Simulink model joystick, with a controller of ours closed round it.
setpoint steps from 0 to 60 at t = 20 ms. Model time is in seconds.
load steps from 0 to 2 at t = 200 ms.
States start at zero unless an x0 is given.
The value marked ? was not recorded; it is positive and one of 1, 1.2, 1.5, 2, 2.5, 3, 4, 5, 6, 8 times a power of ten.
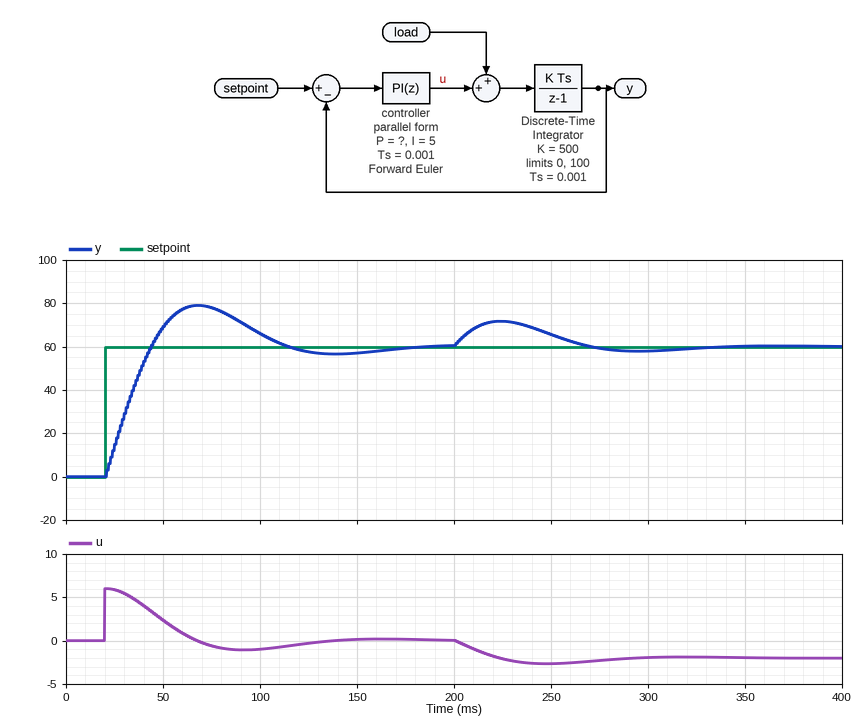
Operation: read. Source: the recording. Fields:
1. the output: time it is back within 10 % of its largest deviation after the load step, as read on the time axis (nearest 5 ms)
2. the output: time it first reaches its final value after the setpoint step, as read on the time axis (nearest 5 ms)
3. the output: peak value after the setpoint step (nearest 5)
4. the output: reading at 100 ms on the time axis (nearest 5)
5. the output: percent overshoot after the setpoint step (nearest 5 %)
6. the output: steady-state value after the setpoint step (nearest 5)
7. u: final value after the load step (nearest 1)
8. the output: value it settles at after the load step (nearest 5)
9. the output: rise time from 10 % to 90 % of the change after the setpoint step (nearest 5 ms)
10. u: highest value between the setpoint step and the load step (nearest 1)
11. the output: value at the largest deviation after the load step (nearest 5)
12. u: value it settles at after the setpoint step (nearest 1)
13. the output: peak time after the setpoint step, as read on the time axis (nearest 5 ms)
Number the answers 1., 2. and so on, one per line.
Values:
1. 320 ms
2. 45 ms
3. 80
4. 65
5. 30 %
6. 60
7. -2
8. 60
9. 20 ms
10. 6
11. 70
12. 0
13. 70 ms
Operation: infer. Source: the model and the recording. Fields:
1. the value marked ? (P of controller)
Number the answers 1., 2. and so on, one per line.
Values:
1. 0.1
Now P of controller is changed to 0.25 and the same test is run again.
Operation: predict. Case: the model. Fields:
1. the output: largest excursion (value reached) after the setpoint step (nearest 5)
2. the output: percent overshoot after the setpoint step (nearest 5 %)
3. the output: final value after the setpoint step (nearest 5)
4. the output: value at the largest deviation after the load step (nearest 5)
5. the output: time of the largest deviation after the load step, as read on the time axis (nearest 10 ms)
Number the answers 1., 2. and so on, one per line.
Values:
1. 65
2. 10 %
3. 60
4. 65
5. 220 ms
